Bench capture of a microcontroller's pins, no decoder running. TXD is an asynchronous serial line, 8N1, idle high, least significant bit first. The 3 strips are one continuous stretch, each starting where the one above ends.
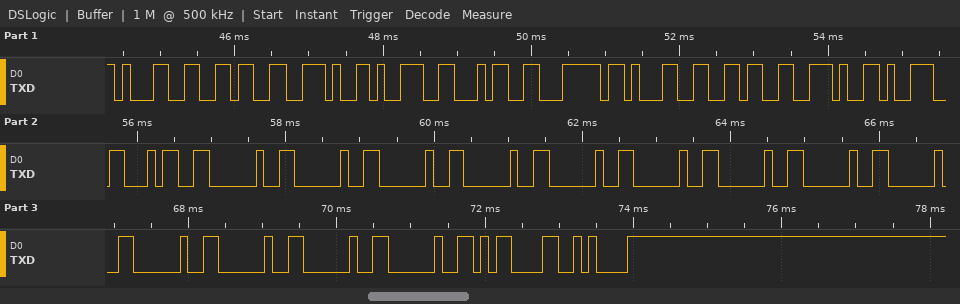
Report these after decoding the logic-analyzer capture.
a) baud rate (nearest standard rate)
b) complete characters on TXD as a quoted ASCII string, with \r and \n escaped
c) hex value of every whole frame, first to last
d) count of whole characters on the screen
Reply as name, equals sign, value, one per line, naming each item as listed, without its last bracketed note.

baud rate = 9600 baud
complete characters on TXD as a quoted ASCII string, with \r and \n escaped = "16.94|16.94             \r\n"
hex value of every whole frame, first to last = 31 36 2E 39 34 7C 31 36 2E 39 34 20 20 20 20 20 20 20 20 20 20 20 20 20 0D 0A
count of whole characters on the screen = 26
